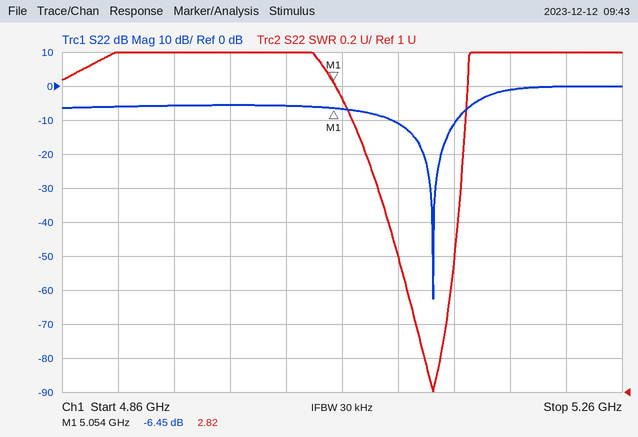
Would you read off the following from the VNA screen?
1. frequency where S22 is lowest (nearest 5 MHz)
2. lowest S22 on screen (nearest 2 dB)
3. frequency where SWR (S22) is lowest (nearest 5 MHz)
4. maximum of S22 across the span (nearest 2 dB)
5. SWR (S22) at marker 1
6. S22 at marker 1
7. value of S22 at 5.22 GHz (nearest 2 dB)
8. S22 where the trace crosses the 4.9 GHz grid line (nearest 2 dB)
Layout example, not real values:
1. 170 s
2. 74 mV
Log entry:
1. 5.125 GHz
2. -62 dB
3. 5.125 GHz
4. 0 dB
5. 2.82
6. -6.45 dB
7. 0 dB
8. -6 dB
